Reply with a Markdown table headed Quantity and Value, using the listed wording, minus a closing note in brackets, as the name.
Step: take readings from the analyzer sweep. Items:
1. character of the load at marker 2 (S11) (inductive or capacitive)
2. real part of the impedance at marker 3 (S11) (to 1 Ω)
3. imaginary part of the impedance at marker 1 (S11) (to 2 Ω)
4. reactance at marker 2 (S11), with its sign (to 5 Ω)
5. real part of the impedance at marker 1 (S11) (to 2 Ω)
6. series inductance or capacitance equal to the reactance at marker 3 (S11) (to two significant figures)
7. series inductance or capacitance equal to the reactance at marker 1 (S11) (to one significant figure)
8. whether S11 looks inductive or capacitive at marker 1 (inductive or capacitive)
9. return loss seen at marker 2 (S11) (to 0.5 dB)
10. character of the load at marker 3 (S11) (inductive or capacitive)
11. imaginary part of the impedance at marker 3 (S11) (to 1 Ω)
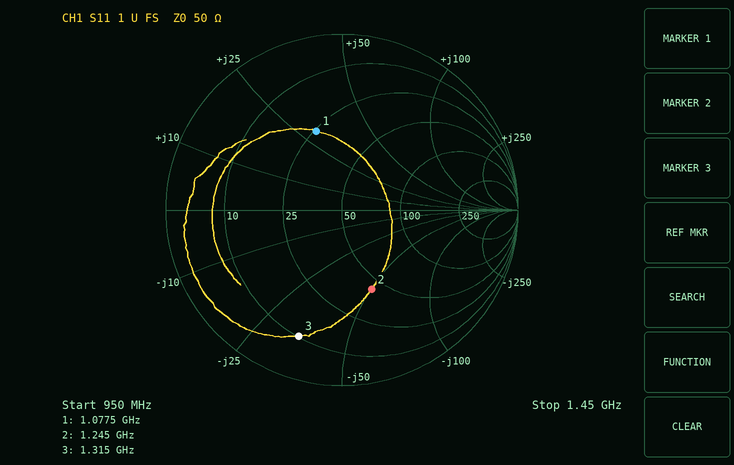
| Quantity | Value |
|---|---|
| character of the load at marker 2 (S11) | capacitive |
| real part of the impedance at marker 3 (S11) | 10 Ω |
| imaginary part of the impedance at marker 1 (S11) | +30 Ω |
| reactance at marker 2 (S11), with its sign | -50 Ω |
| real part of the impedance at marker 1 (S11) | 26 Ω |
| series inductance or capacitance equal to the reactance at marker 3 (S11) | 3.5 pF |
| series inductance or capacitance equal to the reactance at marker 1 (S11) | 4 nH |
| whether S11 looks inductive or capacitive at marker 1 | inductive |
| return loss seen at marker 2 (S11) | 6.5 dB |
| character of the load at marker 3 (S11) | capacitive |
| imaginary part of the impedance at marker 3 (S11) | -35 Ω |
